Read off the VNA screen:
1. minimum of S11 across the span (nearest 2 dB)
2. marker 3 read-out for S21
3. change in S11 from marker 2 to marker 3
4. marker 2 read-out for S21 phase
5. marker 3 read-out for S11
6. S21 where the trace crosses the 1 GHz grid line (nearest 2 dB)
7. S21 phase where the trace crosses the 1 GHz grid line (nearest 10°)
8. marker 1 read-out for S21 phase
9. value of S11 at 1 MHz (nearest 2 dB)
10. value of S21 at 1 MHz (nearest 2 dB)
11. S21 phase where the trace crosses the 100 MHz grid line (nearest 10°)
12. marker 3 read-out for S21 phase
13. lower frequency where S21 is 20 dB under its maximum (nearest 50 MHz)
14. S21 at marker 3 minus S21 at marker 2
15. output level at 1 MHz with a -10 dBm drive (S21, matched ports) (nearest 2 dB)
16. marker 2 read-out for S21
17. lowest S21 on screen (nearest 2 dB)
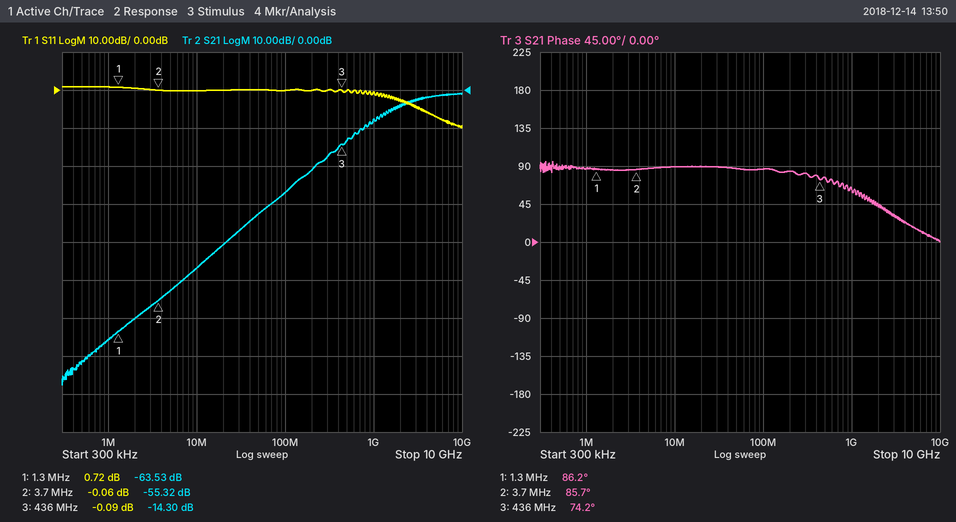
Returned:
-10 dB
-14.30 dB
-0.03 dB
85.7°
-0.09 dB
-8 dB
60°
86.2°
0 dB
-66 dB
90°
74.2°
200 MHz
41.02 dB
-76 dBm
-55.32 dB
-78 dB
